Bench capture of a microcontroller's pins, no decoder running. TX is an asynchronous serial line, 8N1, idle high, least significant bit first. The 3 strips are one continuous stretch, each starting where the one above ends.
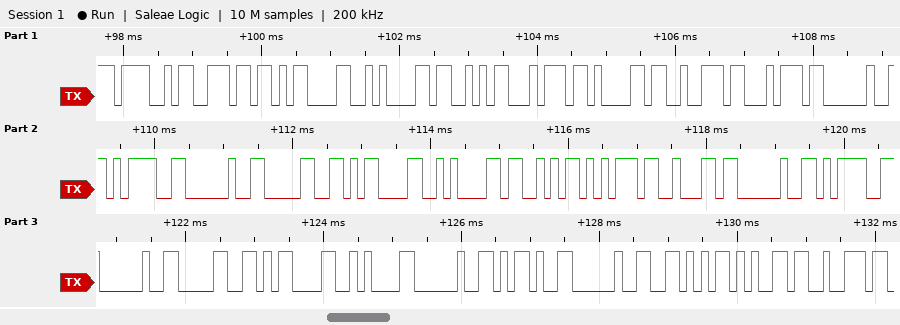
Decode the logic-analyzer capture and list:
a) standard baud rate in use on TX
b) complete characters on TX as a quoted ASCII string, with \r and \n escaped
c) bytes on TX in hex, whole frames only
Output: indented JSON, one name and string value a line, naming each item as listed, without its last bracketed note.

{
  "standard baud rate in use on TX": "9600 baud",
  "complete characters on TX as a quoted ASCII string, with \\r and \\n escaped": "\"On\\r\\nStart = 0\\r\\nSub = 0\\r\\n - Ver\"",
  "bytes on TX in hex, whole frames only": "4F 6E 0D 0A 53 74 61 72 74 20 3D 20 30 0D 0A 53 75 62 20 3D 20 30 0D 0A 20 2D 20 56 65 72"
}
